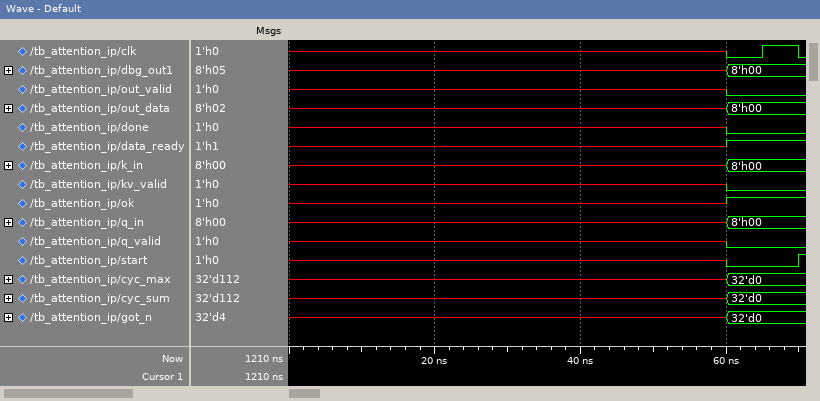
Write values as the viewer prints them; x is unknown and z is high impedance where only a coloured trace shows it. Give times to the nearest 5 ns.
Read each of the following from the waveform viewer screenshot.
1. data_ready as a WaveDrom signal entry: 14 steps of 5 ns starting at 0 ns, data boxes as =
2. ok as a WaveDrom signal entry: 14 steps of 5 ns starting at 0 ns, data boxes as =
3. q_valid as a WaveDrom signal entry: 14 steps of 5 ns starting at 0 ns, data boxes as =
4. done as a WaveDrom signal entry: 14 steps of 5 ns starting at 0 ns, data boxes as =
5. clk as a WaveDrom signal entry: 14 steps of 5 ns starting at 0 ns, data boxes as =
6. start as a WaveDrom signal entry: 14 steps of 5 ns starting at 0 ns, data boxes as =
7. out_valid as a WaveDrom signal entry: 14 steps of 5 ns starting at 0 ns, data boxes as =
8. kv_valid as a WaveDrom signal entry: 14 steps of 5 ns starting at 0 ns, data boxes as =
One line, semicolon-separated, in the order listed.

{name: 'data_ready', wave: 'x...........1.'}; {name: 'ok', wave: 'x...........1.'}; {name: 'q_valid', wave: 'x...........0.'}; {name: 'done', wave: 'x...........0.'}; {name: 'clk', wave: 'x...........01'}; {name: 'start', wave: 'x...........0.'}; {name: 'out_valid', wave: 'x...........0.'}; {name: 'kv_valid', wave: 'x...........0.'}
